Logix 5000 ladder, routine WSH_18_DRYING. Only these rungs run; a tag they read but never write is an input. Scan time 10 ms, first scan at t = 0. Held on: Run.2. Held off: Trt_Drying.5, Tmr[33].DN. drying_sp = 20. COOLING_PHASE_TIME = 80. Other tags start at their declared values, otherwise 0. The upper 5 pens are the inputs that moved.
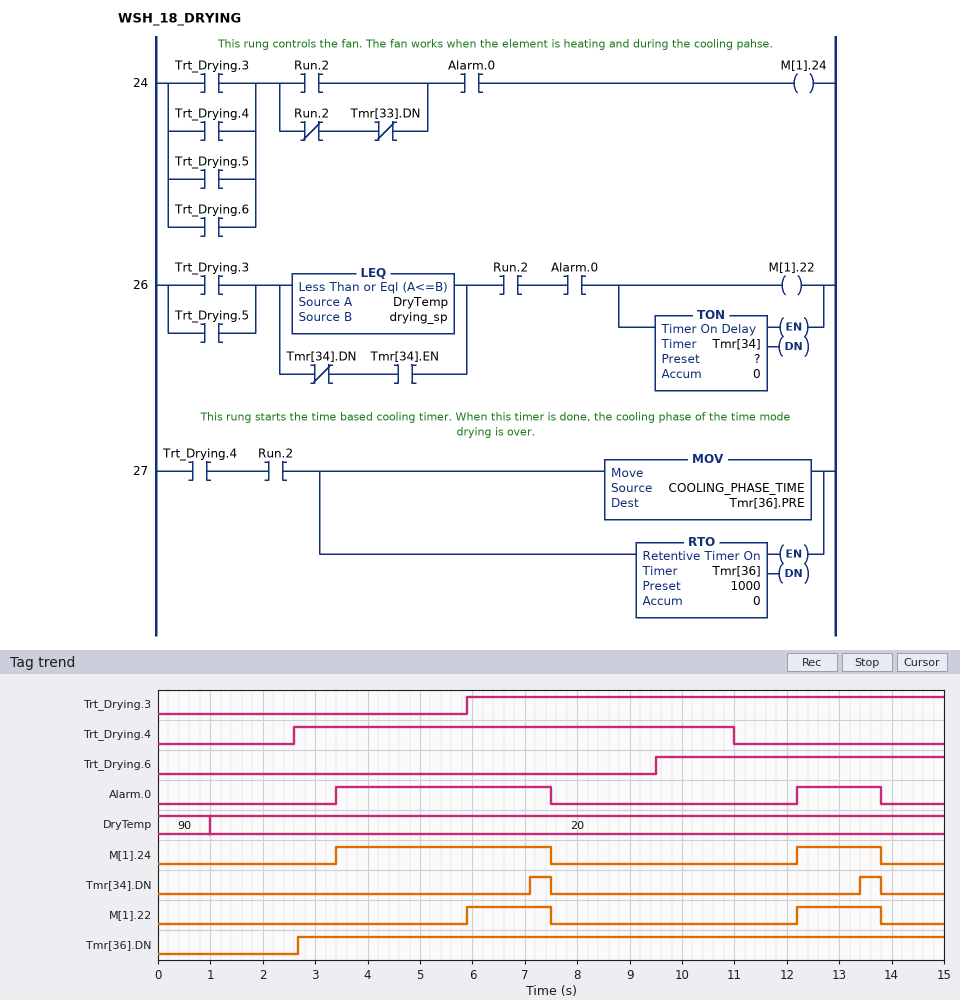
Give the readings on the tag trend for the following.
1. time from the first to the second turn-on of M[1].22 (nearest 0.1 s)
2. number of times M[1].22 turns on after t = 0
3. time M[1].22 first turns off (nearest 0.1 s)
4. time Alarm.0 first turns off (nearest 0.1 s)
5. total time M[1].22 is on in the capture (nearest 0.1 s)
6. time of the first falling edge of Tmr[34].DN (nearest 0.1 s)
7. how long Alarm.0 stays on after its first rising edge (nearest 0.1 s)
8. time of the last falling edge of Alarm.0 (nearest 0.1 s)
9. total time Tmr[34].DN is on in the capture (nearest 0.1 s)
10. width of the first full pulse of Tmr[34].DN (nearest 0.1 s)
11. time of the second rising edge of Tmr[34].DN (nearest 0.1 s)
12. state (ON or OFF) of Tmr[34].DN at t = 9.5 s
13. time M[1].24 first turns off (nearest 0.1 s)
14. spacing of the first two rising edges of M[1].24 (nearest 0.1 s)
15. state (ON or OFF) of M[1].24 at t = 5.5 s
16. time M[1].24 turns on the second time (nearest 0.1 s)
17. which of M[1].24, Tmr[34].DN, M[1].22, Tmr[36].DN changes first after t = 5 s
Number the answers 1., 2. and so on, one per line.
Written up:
1. 6.3 s
2. 2
3. 7.5 s
4. 7.5 s
5. 3.2 s
6. 7.5 s
7. 4.1 s
8. 13.8 s
9. 0.8 s
10. 0.4 s
11. 13.4 s
12. OFF
13. 7.5 s
14. 8.8 s
15. ON
16. 12.2 s
17. M[1].22
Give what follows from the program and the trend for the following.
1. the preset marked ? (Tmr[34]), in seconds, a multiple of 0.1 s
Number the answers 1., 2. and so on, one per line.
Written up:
1. 1.2 s
